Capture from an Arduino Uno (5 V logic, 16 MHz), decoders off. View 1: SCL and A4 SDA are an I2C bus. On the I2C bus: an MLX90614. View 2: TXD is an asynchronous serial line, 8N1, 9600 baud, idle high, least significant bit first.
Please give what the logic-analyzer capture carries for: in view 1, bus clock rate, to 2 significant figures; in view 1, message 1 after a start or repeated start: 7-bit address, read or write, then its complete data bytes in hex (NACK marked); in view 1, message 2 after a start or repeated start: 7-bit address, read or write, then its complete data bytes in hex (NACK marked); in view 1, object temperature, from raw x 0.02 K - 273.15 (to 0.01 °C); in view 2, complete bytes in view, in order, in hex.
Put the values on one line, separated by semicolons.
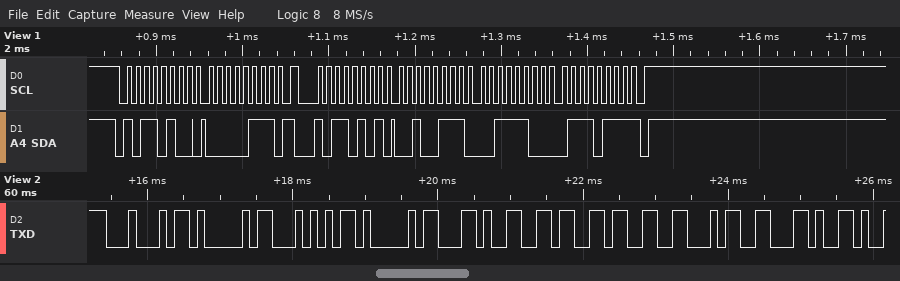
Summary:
100 kHz; 0x5A write: 07; 0x5A read: 27 3C 77 NACK; 34.83 °C; 44 41 54 41 2C 36 33 34 2C
